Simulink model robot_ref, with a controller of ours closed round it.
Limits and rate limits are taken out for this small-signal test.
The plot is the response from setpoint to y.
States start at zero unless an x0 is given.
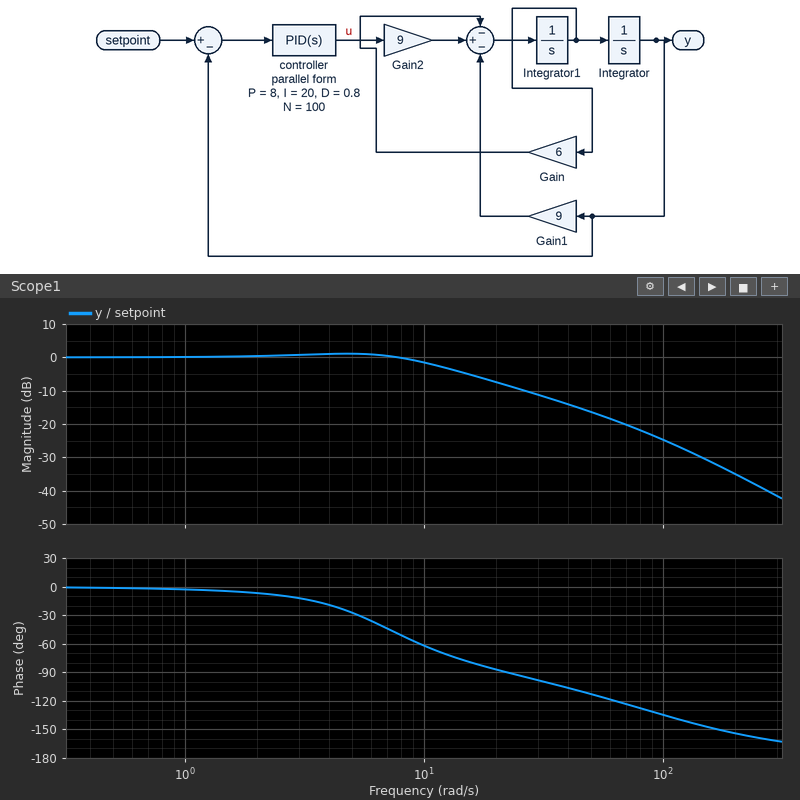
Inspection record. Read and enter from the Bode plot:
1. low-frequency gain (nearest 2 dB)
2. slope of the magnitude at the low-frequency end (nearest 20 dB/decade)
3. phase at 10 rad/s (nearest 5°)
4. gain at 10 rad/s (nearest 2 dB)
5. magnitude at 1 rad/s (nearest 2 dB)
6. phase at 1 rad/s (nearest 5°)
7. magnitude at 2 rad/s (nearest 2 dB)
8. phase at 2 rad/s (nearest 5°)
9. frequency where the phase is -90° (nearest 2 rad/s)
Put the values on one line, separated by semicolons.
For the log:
0 dB; 0 dB/decade; -60°; -2 dB; 0 dB; -5°; 0 dB; -5°; 22 rad/s
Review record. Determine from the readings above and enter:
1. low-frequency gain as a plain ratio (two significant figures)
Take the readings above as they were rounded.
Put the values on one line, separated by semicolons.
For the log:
1.0
